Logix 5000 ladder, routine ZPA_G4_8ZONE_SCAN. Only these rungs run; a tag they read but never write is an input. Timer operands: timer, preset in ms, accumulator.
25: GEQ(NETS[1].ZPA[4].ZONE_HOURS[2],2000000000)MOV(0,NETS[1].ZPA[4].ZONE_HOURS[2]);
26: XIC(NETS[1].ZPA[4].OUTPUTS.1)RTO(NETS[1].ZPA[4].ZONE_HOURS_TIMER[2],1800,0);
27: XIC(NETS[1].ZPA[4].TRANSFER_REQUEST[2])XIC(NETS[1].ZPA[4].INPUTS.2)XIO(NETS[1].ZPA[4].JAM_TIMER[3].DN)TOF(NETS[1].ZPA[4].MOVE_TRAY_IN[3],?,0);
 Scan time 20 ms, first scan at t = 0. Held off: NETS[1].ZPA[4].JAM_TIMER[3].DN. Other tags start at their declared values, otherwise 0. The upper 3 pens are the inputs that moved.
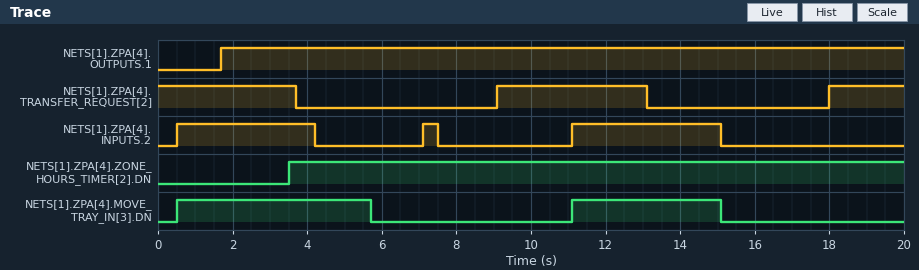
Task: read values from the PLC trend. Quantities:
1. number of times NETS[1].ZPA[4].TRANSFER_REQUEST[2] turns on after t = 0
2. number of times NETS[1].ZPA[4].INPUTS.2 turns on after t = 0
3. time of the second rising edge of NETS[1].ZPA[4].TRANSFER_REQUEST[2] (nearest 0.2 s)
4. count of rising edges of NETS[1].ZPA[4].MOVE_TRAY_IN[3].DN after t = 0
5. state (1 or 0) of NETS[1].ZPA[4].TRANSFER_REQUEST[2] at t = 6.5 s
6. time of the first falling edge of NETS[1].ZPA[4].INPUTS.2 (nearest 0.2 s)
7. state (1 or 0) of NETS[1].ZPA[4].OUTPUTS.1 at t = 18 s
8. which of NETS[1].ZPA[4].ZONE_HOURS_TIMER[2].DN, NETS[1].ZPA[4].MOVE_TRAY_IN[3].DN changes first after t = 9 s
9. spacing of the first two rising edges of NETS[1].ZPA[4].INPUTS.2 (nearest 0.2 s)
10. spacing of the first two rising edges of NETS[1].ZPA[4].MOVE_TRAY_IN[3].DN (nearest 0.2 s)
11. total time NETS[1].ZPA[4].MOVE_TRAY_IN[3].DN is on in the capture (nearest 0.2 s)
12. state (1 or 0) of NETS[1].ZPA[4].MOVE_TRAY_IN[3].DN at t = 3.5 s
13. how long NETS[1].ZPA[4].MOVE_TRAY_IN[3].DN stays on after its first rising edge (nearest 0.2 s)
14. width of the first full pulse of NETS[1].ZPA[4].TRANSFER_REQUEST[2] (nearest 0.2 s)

2
3
18.0 s
2
0
4.2 s
1
NETS[1].ZPA[4].MOVE_TRAY_IN[3].DN
6.6 s
10.6 s
9.2 s
1
5.2 s
4.0 s
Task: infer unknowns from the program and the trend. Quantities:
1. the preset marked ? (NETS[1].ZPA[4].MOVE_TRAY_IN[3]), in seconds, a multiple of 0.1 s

2.0 s
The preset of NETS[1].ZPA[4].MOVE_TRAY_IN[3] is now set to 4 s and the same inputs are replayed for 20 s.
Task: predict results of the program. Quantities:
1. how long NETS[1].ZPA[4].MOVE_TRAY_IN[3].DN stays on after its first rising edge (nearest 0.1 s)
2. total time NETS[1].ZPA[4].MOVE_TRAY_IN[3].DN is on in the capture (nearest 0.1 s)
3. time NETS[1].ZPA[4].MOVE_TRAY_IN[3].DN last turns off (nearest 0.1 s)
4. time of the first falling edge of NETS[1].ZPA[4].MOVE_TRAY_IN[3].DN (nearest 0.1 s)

7.2 s
13.2 s
17.1 s
7.7 s
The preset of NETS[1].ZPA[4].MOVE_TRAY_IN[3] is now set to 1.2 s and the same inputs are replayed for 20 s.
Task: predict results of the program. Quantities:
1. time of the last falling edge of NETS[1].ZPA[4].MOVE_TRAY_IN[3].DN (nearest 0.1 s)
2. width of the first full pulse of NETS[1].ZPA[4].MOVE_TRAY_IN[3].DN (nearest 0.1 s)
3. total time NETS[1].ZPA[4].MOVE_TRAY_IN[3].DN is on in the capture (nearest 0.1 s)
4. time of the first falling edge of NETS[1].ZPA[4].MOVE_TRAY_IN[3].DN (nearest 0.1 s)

14.3 s
4.4 s
7.6 s
4.9 s
